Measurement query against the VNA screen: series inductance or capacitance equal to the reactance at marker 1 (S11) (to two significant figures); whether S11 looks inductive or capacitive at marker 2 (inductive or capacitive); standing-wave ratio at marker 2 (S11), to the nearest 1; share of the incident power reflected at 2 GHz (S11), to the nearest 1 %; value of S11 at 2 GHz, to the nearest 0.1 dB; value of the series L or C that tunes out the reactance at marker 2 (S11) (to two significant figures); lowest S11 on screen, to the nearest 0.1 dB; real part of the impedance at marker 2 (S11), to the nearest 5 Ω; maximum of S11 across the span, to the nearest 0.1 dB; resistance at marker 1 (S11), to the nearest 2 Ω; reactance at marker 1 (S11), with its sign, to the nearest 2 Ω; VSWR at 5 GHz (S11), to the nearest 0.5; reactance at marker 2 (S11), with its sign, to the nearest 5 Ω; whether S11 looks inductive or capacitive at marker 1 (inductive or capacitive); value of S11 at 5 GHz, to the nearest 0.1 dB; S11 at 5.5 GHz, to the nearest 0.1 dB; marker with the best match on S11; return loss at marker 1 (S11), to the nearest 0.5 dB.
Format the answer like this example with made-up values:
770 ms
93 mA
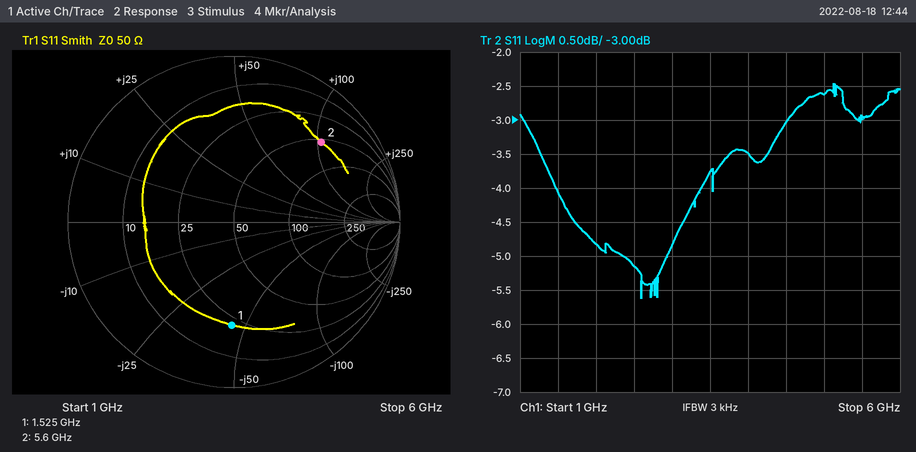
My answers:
2.4 pF
inductive
6
33 %
-4.8 dB
270 fF
-5.6 dB
55 Ω
-2.5 dB
22 Ω
-44 Ω
6.5
+105 Ω
capacitive
-2.6 dB
-3.0 dB
marker 1
4.0 dB
